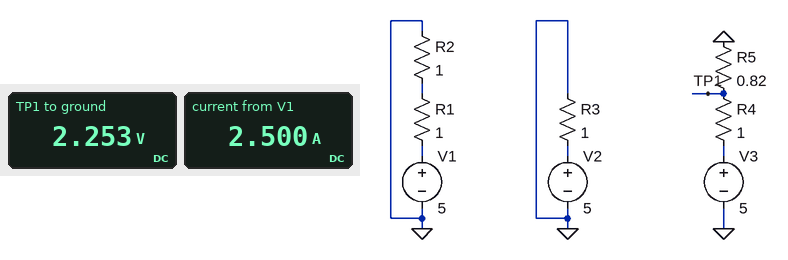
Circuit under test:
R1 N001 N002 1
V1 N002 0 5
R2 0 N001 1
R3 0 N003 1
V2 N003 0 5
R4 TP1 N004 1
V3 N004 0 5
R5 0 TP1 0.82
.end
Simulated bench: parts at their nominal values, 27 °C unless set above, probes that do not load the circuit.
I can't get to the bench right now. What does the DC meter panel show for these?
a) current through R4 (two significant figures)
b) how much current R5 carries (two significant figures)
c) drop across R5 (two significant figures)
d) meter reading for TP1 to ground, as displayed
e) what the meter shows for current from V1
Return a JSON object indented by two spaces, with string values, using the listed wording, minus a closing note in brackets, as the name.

{
  "current through R4": "2.7 A",
  "how much current R5 carries": "2.7 A",
  "drop across R5": "2.3 V",
  "meter reading for TP1 to ground, as displayed": "2.253 V",
  "what the meter shows for current from V1": "2.500 A"
}
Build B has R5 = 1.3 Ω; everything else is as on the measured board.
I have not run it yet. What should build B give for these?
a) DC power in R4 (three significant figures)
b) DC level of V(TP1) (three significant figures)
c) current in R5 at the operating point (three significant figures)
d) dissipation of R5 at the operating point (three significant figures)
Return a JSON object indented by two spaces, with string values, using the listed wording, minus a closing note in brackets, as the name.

{
  "DC power in R4": "4.73 W",
  "DC level of V(TP1)": "2.83 V",
  "current in R5 at the operating point": "2.17 A",
  "dissipation of R5 at the operating point": "6.14 W"
}
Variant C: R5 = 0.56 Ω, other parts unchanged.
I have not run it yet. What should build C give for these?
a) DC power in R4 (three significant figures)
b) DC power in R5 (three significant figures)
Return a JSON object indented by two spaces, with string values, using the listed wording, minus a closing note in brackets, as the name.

{
  "DC power in R4": "10.3 W",
  "DC power in R5": "5.75 W"
}
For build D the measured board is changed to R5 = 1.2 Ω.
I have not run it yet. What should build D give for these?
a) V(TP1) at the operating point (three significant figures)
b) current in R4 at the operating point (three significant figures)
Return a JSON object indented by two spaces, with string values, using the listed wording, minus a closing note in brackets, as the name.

{
  "V(TP1) at the operating point": "2.73 V",
  "current in R4 at the operating point": "2.27 A"
}
